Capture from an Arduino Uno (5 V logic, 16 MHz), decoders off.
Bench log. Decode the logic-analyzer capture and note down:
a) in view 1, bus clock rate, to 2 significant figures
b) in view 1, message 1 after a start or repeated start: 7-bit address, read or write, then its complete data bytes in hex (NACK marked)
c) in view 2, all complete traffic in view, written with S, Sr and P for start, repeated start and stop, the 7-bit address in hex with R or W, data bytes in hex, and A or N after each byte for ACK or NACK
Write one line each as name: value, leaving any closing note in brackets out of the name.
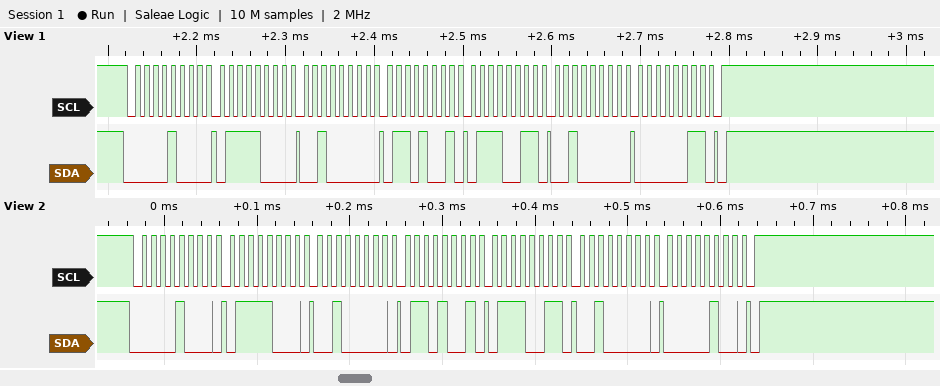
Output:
in view 1, bus clock rate, to 2 significant figures: 100 kHz
in view 1, message 1 after a start or repeated start: 7-bit address, read or write, then its complete data bytes in hex: 0x04 write: 78 20 69 73 20 03
in view 2, all complete traffic in view, written with S, Sr and P for start, repeated start and stop, the 7-bit address in hex with R or W, data bytes in hex, and A or N after each byte for ACK or NACK: S 04W A 78 A 20 A 69 A 73 A 20 A 04 A P
